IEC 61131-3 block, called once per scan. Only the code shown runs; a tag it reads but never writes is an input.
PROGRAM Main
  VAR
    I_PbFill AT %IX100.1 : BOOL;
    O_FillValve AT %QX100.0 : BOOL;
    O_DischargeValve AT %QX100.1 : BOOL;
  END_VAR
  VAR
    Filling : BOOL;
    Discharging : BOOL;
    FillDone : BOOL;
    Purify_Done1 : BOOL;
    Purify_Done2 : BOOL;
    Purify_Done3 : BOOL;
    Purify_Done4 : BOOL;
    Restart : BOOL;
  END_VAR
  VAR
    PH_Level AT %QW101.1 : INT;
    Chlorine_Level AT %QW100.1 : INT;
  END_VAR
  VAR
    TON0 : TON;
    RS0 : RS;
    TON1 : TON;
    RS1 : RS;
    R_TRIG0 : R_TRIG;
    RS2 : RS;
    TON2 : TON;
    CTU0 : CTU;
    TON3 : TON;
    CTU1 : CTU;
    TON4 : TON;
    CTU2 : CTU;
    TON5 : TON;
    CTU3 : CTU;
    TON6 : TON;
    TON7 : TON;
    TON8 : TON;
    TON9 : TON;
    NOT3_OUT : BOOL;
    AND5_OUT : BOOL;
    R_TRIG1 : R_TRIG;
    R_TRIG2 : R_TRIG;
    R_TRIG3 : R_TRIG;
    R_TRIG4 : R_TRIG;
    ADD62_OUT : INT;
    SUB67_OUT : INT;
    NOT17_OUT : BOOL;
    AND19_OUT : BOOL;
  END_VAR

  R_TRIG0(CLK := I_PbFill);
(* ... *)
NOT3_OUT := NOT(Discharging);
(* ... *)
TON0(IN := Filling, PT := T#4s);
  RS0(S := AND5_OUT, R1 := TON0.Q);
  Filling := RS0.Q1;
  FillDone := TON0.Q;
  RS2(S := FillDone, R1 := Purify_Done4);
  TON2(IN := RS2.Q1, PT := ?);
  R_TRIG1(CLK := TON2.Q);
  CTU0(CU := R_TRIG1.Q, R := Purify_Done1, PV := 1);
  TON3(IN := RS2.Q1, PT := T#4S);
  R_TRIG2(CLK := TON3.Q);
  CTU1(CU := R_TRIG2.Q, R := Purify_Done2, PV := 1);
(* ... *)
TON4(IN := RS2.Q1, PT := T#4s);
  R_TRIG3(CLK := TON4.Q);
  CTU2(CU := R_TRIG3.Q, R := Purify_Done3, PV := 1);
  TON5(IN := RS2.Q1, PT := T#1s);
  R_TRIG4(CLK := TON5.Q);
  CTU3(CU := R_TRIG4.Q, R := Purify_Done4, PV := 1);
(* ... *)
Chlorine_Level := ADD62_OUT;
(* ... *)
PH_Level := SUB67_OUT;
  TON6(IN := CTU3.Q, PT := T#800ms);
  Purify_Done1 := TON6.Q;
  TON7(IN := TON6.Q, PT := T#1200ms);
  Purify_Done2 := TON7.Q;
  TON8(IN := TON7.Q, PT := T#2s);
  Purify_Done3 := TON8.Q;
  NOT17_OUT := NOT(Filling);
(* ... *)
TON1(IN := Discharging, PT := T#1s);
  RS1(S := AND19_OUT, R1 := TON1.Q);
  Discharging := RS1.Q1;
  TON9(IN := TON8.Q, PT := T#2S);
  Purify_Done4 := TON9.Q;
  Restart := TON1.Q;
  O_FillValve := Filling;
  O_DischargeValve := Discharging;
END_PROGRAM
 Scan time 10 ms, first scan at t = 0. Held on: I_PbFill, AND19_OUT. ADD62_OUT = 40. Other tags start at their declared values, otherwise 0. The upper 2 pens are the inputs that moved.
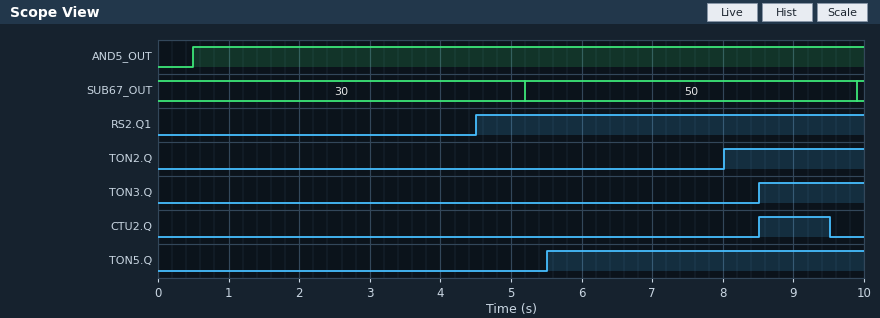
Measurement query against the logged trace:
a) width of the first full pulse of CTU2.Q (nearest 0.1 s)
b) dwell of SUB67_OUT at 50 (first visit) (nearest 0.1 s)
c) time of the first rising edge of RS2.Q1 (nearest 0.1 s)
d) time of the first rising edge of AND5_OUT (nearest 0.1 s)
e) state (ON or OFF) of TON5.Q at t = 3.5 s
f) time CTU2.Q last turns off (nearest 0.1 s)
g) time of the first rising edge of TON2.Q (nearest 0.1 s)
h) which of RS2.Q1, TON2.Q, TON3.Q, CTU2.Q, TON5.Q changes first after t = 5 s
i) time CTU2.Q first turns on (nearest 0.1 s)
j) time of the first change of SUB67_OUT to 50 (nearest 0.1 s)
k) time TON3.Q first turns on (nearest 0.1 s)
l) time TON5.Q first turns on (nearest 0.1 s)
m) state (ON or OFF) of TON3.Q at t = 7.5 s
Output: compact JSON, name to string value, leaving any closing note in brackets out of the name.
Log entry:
{"width of the first full pulse of CTU2.Q": "1.0 s", "dwell of SUB67_OUT at 50 (first visit)": "4.7 s", "time of the first rising edge of RS2.Q1": "4.5 s", "time of the first rising edge of AND5_OUT": "0.5 s", "state (ON or OFF) of TON5.Q at t = 3.5 s": "OFF", "time CTU2.Q last turns off": "9.5 s", "time of the first rising edge of TON2.Q": "8.0 s", "which of RS2.Q1, TON2.Q, TON3.Q, CTU2.Q, TON5.Q changes first after t = 5 s": "TON5.Q", "time CTU2.Q first turns on": "8.5 s", "time of the first change of SUB67_OUT to 50": "5.2 s", "time TON3.Q first turns on": "8.5 s", "time TON5.Q first turns on": "5.5 s", "state (ON or OFF) of TON3.Q at t = 7.5 s": "OFF"}
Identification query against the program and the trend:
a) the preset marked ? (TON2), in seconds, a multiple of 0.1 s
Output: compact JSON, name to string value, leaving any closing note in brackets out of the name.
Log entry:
{"the preset marked ? (TON2), in seconds, a multiple of 0.1 s": "3.5 s"}
